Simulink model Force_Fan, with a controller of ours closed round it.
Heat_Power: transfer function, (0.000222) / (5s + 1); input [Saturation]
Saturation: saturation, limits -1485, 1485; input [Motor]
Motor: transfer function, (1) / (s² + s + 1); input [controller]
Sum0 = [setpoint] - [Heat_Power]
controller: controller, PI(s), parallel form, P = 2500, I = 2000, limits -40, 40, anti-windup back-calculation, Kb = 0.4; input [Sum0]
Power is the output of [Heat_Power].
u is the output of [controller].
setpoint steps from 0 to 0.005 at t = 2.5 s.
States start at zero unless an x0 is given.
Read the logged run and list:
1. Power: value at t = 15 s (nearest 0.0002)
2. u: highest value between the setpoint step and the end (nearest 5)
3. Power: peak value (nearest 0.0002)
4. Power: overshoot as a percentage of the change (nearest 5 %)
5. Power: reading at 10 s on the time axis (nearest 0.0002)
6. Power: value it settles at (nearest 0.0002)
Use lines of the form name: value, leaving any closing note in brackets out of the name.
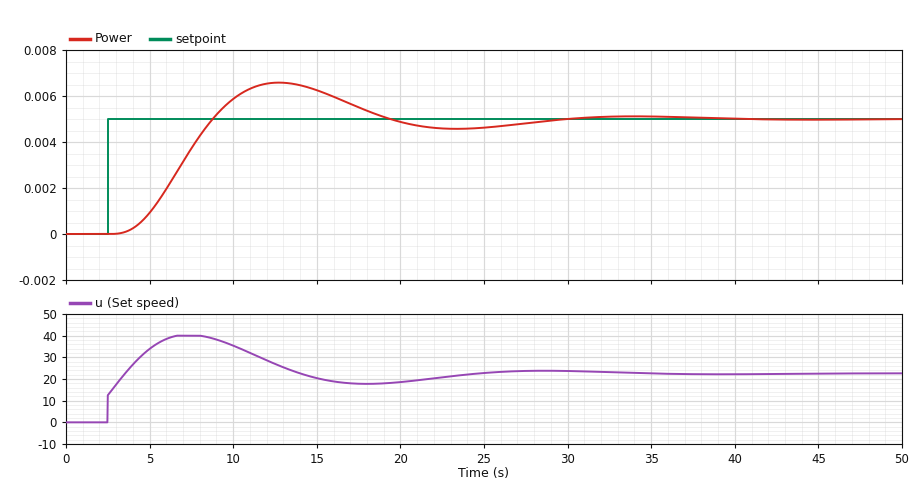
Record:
Power: value at t = 15 s: 0.0062
u: highest value between the setpoint step and the end: 40
Power: peak value: 0.0066
Power: overshoot as a percentage of the change: 30 %
Power: reading at 10 s on the time axis: 0.0058
Power: value it settles at: 0.0050
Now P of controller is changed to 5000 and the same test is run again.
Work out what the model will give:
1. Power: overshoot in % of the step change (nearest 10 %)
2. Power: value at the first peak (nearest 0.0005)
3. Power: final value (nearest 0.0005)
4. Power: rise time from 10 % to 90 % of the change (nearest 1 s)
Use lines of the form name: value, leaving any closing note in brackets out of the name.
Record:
Power: overshoot in % of the step change: 20 %
Power: value at the first peak: 0.0060
Power: final value: 0.0050
Power: rise time from 10 % to 90 % of the change: 3 s
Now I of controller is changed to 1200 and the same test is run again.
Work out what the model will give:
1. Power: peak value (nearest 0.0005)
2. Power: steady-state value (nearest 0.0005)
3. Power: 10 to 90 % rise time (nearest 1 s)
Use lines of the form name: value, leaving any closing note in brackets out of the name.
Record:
Power: peak value: 0.0055
Power: steady-state value: 0.0050
Power: 10 to 90 % rise time: 6 s
